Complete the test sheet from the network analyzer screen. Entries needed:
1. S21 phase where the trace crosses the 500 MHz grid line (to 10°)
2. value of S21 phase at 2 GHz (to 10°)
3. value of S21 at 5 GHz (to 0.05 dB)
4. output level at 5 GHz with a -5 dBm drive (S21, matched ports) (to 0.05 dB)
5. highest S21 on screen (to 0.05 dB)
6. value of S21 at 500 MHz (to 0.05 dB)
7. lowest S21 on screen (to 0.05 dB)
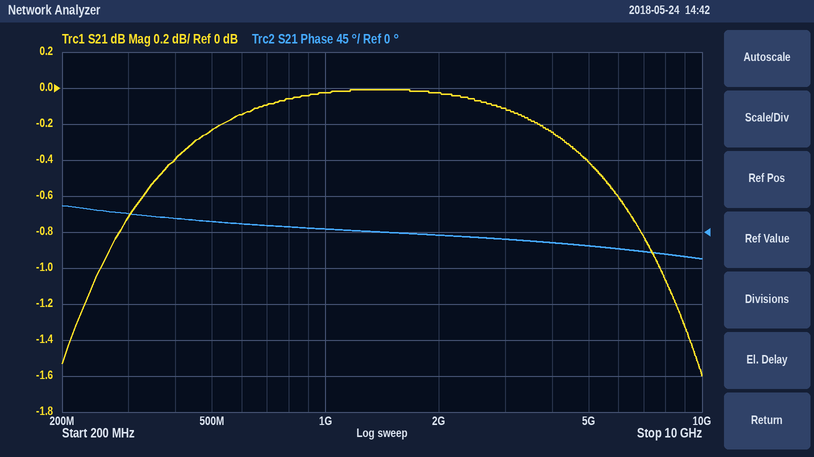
10°
0°
-0.40 dB
-5.40 dBm
0.00 dB
-0.25 dB
-1.60 dB
